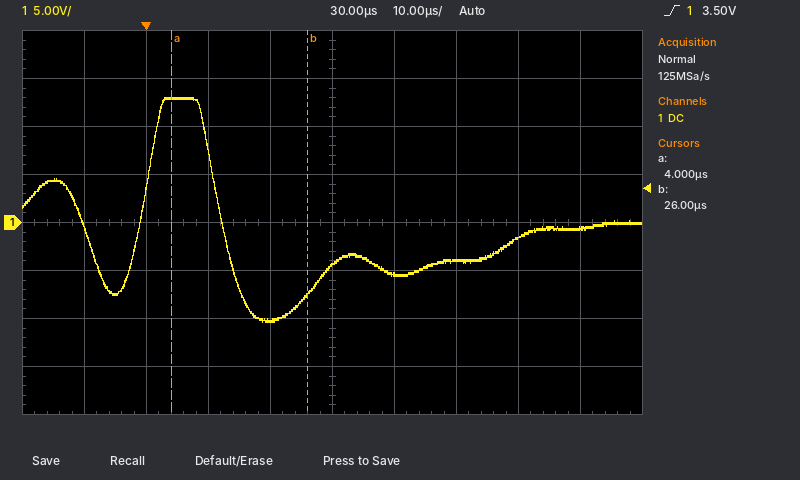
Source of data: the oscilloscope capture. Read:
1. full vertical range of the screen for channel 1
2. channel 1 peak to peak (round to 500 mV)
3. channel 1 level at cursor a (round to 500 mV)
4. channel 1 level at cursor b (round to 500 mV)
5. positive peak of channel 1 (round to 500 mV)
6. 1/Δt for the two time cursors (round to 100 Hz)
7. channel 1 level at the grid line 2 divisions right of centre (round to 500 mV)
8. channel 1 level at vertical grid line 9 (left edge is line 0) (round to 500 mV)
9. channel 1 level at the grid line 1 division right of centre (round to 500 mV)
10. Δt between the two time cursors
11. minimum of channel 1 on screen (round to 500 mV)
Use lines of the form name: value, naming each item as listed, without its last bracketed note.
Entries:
full vertical range of the screen for channel 1: 40 V
channel 1 peak to peak: 23.5 V
channel 1 level at cursor a: 13.0 V
channel 1 level at cursor b: -7.5 V
positive peak of channel 1: 13.0 V
1/Δt for the two time cursors: 45.5 kHz
channel 1 level at the grid line 2 divisions right of centre: -4.0 V
channel 1 level at vertical grid line 9 (left edge is line 0): -500 mV
channel 1 level at the grid line 1 division right of centre: -5.5 V
Δt between the two time cursors: 22 µs
minimum of channel 1 on screen: -10.5 V
